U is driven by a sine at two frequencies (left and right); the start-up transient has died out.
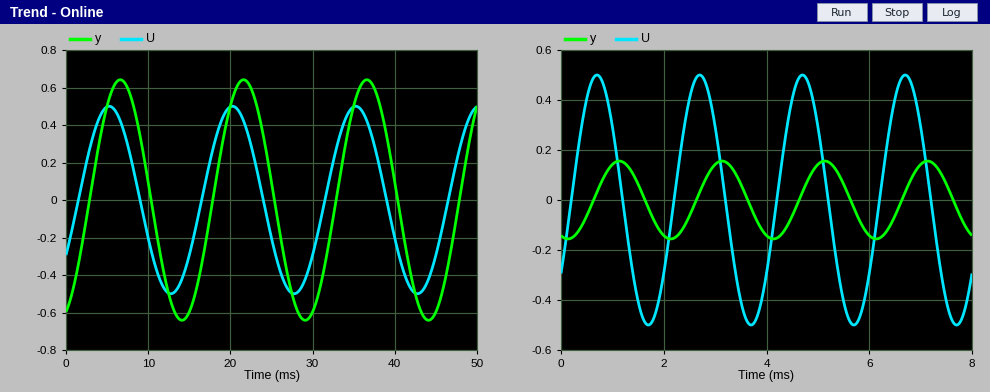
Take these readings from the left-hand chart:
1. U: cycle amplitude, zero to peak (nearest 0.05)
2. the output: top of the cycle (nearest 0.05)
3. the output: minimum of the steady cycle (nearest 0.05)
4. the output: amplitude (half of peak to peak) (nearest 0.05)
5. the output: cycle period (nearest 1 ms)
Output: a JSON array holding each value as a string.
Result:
["0.50", "0.65", "-0.65", "0.65", "15 ms"]
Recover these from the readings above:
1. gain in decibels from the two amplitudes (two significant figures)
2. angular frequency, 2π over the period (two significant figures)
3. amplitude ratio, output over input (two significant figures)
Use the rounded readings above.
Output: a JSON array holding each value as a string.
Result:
["2.3 dB", "0.42 rad/ms", "1.3"]
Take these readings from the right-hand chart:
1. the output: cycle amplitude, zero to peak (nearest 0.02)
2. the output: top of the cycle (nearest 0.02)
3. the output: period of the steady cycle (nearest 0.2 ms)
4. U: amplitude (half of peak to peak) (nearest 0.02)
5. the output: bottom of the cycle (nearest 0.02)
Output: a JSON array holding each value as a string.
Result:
["0.16", "0.16", "2.0 ms", "0.50", "-0.16"]
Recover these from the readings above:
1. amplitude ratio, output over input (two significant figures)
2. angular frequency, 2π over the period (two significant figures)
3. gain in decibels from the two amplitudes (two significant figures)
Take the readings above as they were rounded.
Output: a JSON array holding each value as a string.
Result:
["0.32", "3.1 rad/ms", "-9.9 dB"]
